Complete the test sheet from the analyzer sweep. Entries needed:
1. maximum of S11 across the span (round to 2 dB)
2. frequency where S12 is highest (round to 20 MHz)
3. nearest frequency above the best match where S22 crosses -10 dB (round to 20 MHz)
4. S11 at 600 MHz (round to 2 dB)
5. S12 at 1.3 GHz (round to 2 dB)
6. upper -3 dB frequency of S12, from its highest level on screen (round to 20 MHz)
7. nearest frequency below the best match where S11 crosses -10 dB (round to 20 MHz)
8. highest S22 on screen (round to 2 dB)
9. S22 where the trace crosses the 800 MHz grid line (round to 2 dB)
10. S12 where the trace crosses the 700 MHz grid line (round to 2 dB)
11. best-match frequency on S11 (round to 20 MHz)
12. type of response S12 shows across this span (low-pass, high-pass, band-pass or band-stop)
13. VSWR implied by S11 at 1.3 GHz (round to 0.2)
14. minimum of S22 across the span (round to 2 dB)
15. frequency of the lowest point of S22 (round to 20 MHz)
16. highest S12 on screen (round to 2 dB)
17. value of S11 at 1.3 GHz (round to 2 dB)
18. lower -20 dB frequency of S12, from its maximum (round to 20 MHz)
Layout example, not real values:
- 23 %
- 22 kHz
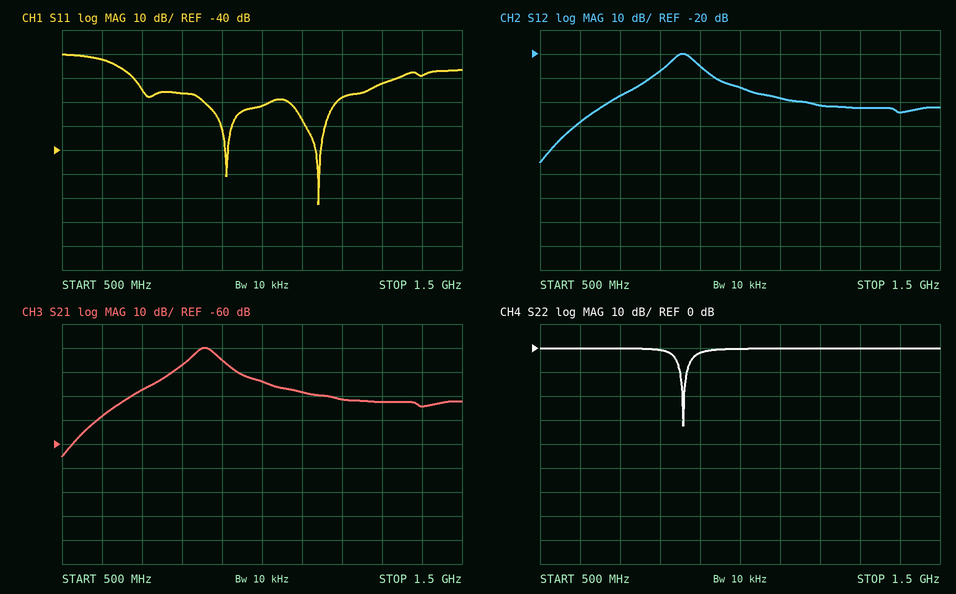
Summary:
- 0 dB
- 860 MHz
- 860 MHz
- -2 dB
- -42 dB
- 880 MHz
- 680 MHz
- 0 dB
- 0 dB
- -38 dB
- 1.14 GHz
- band-pass
- 1.6
- -32 dB
- 860 MHz
- -20 dB
- -12 dB
- 680 MHz
